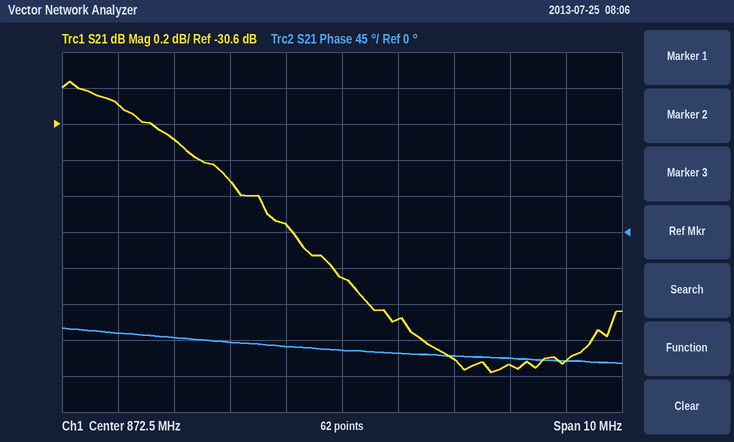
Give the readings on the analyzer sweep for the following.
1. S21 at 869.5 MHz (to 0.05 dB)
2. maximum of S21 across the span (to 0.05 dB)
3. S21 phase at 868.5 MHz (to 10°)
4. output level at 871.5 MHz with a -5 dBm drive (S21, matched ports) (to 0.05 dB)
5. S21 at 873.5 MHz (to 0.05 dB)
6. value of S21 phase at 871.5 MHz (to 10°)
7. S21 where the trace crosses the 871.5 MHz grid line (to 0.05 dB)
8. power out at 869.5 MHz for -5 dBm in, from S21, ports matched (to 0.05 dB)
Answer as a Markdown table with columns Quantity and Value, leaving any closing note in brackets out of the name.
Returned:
| Quantity | Value |
|---|---|
| S21 at 869.5 MHz | -30.70 dB |
| maximum of S21 across the span | -30.35 dB |
| S21 phase at 868.5 MHz | -130° |
| output level at 871.5 MHz with a -5 dBm drive (S21, matched ports) | -36.15 dBm |
| S21 at 873.5 MHz | -31.70 dB |
| value of S21 phase at 871.5 MHz | -140° |
| S21 where the trace crosses the 871.5 MHz grid line | -31.15 dB |
| power out at 869.5 MHz for -5 dBm in, from S21, ports matched | -35.70 dBm |
